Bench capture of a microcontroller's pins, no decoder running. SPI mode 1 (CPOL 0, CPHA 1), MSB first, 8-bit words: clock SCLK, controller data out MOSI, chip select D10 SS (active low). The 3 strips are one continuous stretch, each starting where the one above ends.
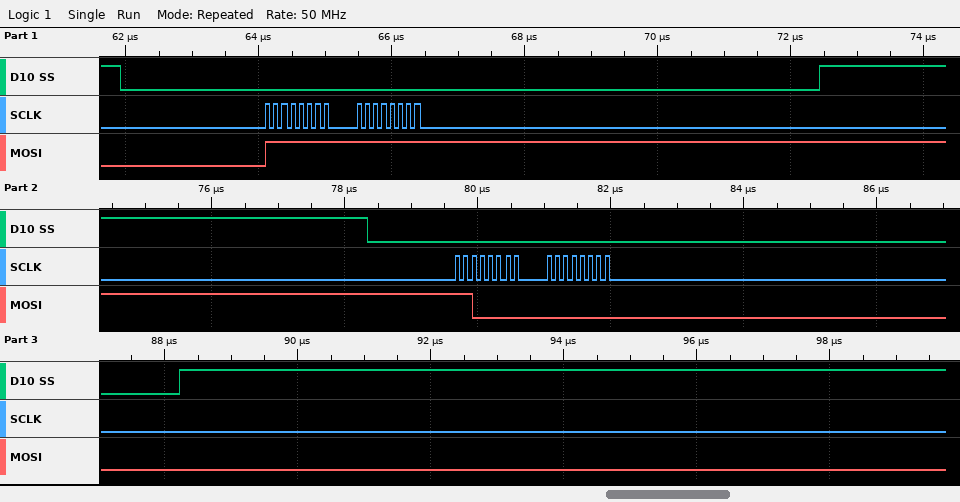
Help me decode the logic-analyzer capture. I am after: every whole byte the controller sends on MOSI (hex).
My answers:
0xFF 0xFF 0xC0 0x00
